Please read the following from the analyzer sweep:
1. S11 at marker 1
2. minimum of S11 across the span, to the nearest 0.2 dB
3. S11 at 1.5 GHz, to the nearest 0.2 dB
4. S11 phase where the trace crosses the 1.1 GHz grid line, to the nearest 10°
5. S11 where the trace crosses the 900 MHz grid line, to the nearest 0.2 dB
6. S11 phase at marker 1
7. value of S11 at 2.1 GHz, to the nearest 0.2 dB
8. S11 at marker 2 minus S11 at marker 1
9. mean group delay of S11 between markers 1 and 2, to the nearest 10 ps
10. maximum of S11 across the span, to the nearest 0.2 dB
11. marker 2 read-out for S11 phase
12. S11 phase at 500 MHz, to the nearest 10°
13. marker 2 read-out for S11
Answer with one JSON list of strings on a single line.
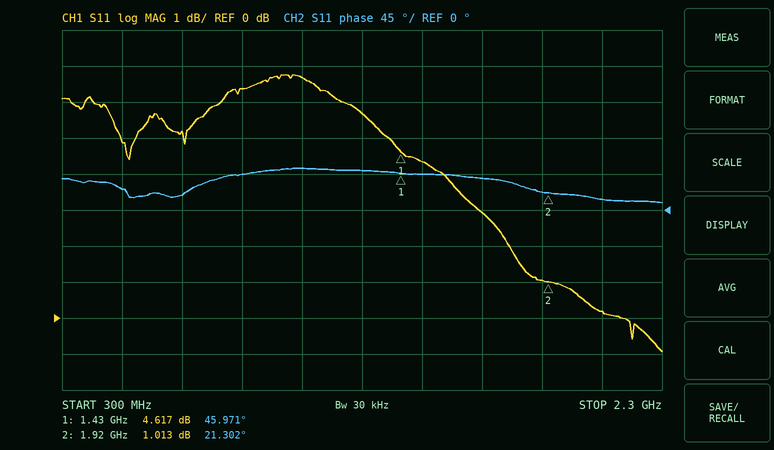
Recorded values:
["4.617 dB", "-1.0 dB", "4.4 dB", "50°", "6.4 dB", "45.971°", "0.2 dB", "-3.604 dB", "140 ps", "6.8 dB", "21.302°", "30°", "1.013 dB"]
